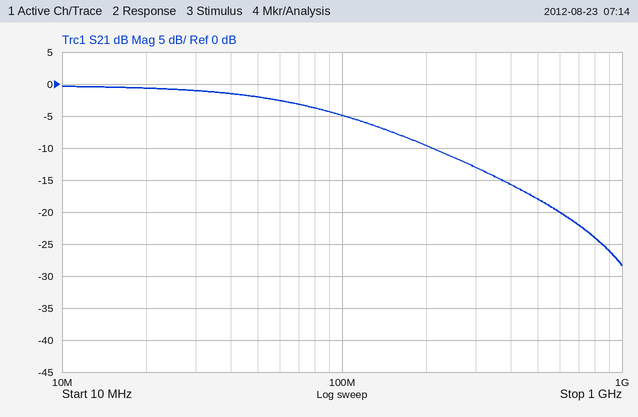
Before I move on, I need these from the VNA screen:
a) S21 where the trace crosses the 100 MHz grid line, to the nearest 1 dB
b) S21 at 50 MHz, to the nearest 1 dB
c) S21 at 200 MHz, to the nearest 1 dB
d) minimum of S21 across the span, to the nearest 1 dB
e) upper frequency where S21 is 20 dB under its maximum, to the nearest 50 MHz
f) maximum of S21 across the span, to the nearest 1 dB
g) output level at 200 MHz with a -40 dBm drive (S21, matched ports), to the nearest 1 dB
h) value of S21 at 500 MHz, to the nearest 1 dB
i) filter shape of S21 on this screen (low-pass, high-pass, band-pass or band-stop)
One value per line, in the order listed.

-5 dB
-2 dB
-10 dB
-28 dB
600 MHz
0 dB
-50 dBm
-18 dB
low-pass
